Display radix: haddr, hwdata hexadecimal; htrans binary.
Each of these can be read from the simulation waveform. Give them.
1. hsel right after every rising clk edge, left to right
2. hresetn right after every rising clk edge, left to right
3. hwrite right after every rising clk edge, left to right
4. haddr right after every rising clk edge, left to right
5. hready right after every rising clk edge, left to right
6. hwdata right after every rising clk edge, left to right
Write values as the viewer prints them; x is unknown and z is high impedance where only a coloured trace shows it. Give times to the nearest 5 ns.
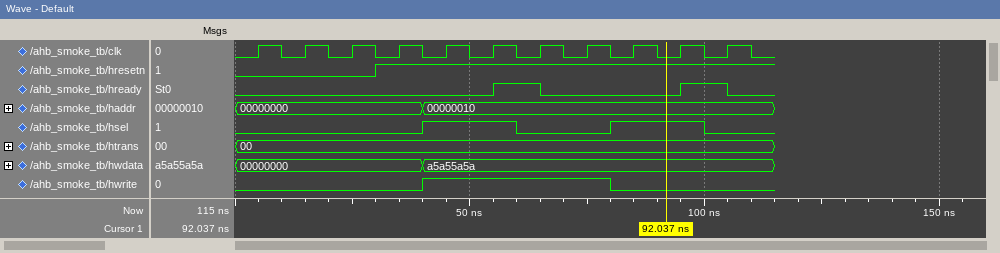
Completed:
0 0 0 0 1 1 0 0 1 1 0
0 0 0 1 1 1 1 1 1 1 1
0 0 0 0 1 1 1 1 0 0 0
00000000, 00000000, 00000000, 00000000, 00000010, 00000010, 00000010, 00000010, 00000010, 00000010, 00000010
0 0 0 0 0 1 0 0 0 1 0
00000000, 00000000, 00000000, 00000000, a5a55a5a, a5a55a5a, a5a55a5a, a5a55a5a, a5a55a5a, a5a55a5a, a5a55a5a
